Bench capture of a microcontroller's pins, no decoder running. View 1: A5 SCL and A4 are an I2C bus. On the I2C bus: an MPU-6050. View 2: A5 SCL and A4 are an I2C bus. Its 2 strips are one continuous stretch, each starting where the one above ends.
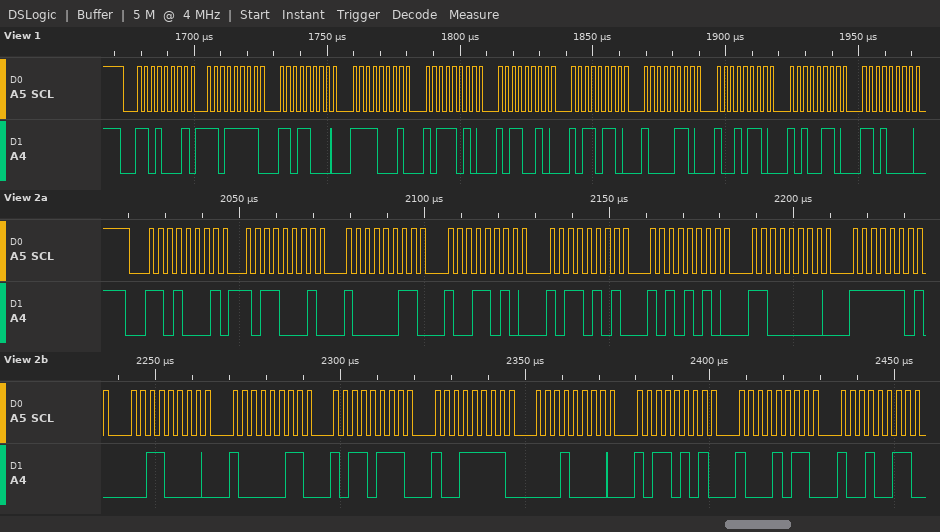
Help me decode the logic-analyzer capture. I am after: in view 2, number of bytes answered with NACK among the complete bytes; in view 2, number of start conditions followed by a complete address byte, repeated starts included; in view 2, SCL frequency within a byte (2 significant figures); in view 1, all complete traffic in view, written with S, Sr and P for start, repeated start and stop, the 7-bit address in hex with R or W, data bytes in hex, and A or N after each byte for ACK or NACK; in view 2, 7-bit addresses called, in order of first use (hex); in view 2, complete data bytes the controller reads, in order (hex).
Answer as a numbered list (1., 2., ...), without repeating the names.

1. 0
2. 1
3. 400 kHz
4. S 68R A DF A D8 A F1 A BA A B2 A B6 A 86 A 96 A A6 A D0 A
5. 0x68
6. B1 83 9A B5 AA C0 FD 30 83 B7 9F 10 B5 8B 93
